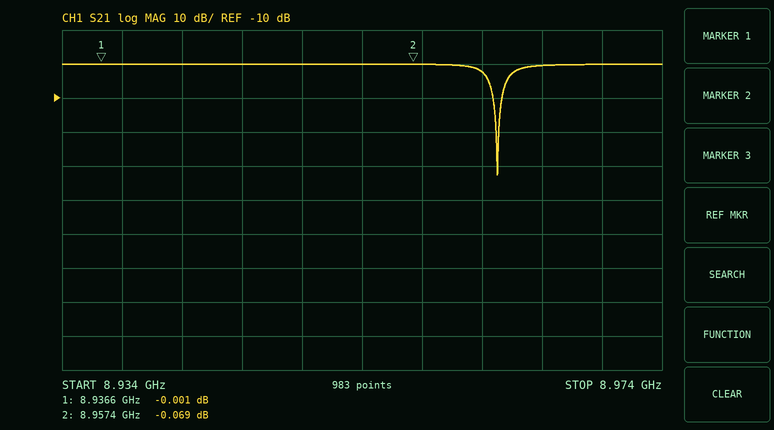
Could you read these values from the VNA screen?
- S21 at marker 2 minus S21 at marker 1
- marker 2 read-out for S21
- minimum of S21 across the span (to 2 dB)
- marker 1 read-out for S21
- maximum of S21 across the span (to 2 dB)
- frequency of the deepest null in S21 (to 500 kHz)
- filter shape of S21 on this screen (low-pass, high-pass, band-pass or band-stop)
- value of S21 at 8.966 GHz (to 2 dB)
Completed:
-0.068 dB
-0.069 dB
-32 dB
-0.001 dB
0 dB
8.9630 GHz
band-stop
0 dB
